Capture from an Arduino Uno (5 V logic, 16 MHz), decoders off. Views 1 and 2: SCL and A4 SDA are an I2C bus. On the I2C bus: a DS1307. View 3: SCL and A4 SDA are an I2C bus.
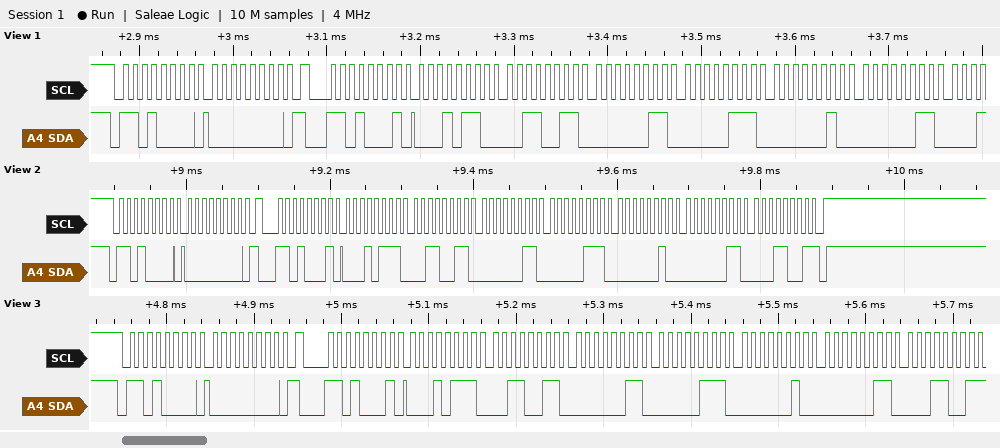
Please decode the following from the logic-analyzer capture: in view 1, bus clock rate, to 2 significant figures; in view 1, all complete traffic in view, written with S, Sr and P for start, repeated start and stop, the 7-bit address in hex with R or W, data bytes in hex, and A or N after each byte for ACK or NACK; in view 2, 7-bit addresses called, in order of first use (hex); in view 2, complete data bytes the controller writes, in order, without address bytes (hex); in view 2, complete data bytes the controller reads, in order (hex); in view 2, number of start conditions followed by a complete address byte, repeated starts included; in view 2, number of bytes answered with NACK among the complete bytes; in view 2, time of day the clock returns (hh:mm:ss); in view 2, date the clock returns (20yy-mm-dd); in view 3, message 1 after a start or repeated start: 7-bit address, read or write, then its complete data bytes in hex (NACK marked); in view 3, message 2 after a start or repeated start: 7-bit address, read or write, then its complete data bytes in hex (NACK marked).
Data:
100 kHz
S 68W A 00 A Sr 68R A 16 A 33 A 03 A 07 A 02 A 03 A
0x68
00
17 33 03 07 02 03 19
2
1
03:33:17
2019-03-02
0x68 write: 00
0x68 read: 17 33 03 07 02 03 19 NACK
